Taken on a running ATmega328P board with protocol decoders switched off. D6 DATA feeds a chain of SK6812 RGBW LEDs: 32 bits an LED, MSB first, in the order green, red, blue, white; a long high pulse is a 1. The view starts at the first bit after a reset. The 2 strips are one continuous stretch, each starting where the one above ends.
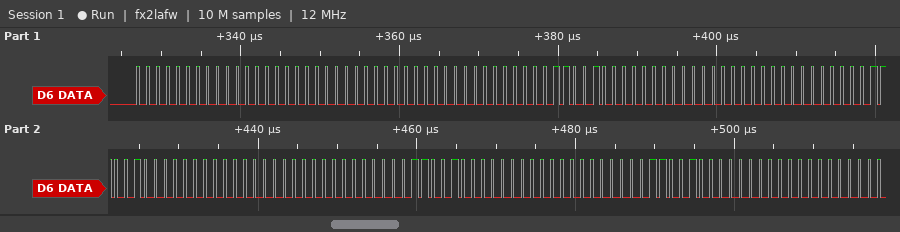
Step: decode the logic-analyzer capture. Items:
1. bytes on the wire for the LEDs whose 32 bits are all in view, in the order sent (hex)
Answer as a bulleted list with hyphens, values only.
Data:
- 00 00 00 00 00 32 00 00 00 32 00 00 00 32 00 00
